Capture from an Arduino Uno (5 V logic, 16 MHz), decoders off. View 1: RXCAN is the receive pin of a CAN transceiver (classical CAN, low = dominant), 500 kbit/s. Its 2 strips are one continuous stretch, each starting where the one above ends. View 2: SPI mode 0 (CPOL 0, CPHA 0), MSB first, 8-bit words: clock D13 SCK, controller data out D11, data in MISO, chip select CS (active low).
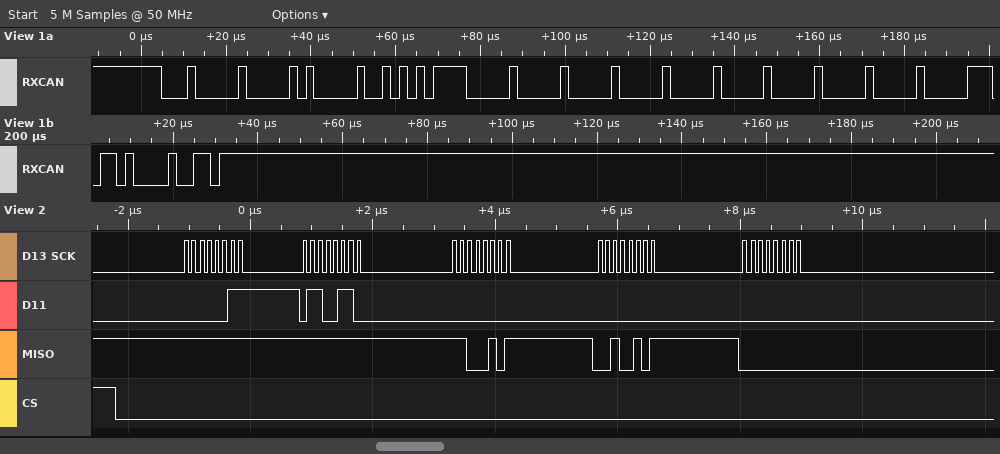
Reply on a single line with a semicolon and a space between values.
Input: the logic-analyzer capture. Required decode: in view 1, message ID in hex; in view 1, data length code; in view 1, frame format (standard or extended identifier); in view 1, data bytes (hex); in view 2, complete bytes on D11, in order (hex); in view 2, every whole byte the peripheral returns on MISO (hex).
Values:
0x100; 8; standard; 0A BC 00 00 00 00 00 00; 03 66 00 00 00; FF FF C5 25 00
